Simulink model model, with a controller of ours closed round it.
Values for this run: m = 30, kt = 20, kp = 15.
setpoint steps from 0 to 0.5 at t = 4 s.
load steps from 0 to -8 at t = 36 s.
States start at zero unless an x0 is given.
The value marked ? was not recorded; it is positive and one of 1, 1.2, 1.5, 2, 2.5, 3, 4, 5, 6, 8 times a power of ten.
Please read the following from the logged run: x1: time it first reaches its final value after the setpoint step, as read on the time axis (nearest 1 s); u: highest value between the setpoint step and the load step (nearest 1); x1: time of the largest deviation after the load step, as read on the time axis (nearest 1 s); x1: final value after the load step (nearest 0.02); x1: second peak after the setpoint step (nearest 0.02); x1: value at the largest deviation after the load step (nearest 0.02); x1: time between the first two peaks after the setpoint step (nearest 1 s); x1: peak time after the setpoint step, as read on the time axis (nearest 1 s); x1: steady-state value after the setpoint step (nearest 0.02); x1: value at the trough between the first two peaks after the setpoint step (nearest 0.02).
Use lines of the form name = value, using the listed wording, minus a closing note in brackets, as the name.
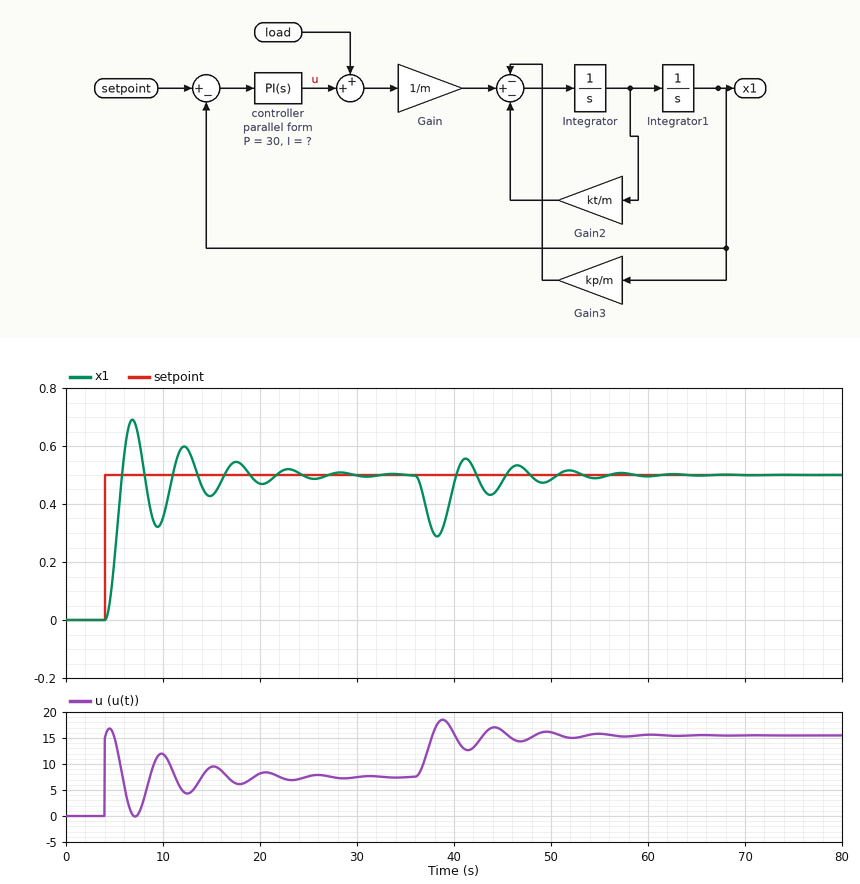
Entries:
x1: time it first reaches its final value after the setpoint step, as read on the time axis = 6 s
u: highest value between the setpoint step and the load step = 17
x1: time of the largest deviation after the load step, as read on the time axis = 38 s
x1: final value after the load step = 0.50
x1: second peak after the setpoint step = 0.60
x1: value at the largest deviation after the load step = 0.28
x1: time between the first two peaks after the setpoint step = 5 s
x1: peak time after the setpoint step, as read on the time axis = 7 s
x1: steady-state value after the setpoint step = 0.50
x1: value at the trough between the first two peaks after the setpoint step = 0.32
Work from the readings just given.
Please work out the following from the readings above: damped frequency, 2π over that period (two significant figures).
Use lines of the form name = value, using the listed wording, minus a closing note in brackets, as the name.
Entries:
damped frequency, 2π over that period = 1.3 rad/s
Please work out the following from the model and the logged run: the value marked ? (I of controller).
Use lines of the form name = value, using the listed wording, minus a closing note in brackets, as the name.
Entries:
the value marked ? = 15
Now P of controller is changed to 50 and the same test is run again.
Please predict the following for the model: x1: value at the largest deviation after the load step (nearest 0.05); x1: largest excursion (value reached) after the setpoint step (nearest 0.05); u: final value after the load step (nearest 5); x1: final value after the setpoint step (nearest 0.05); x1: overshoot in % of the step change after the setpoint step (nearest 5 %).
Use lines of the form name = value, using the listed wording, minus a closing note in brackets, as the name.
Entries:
x1: value at the largest deviation after the load step = 0.35
x1: largest excursion (value reached) after the setpoint step = 0.70
u: final value after the load step = 15
x1: final value after the setpoint step = 0.50
x1: overshoot in % of the step change after the setpoint step = 40 %
